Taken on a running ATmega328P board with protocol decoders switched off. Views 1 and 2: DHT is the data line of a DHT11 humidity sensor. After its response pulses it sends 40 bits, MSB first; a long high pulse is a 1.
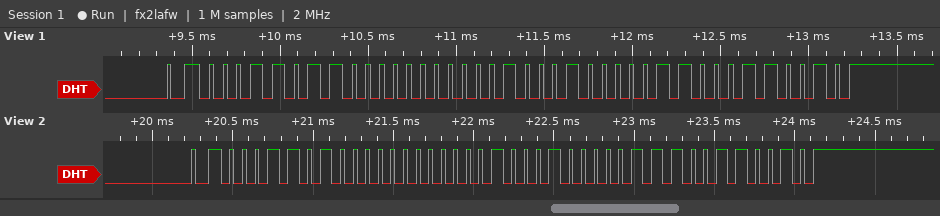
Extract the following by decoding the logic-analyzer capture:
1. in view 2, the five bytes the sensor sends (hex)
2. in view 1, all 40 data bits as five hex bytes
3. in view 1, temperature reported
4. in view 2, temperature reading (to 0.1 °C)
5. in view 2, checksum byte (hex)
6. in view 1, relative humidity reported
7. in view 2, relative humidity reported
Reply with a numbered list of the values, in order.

1. 1A 00 11 07 32
2. 1B 00 11 06 32
3. 17.6 °C
4. 17.7 °C
5. 0x32
6. 27 %
7. 26 %
